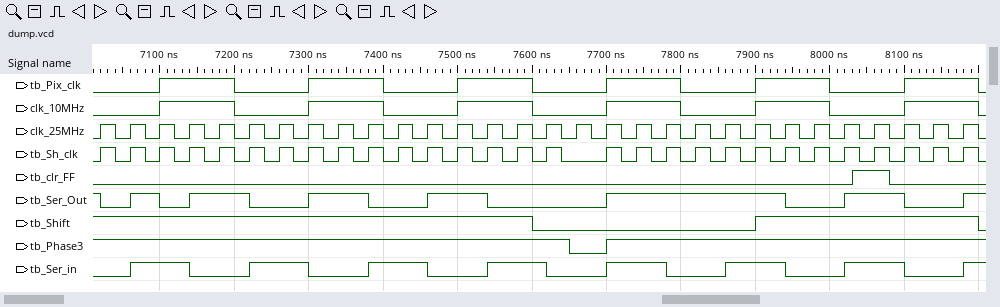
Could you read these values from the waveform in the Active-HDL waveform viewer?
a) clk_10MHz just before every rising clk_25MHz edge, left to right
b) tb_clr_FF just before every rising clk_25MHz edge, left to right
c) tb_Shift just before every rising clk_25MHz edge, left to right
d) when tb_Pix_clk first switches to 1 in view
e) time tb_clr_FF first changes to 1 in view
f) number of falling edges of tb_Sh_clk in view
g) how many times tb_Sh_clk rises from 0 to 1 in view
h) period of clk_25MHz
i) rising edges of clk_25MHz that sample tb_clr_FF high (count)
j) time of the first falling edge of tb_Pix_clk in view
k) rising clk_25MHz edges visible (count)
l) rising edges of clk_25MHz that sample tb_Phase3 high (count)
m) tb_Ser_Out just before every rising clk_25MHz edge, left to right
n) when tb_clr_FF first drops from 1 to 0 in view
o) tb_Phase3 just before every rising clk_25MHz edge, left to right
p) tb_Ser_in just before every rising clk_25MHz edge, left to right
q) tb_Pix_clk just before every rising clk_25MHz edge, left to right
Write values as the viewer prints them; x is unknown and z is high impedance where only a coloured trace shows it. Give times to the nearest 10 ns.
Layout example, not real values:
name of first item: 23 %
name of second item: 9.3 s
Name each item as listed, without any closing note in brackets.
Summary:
clk_10MHz just before every rising clk_25MHz edge, left to right: 0 0 0 1 1 0 0 0 1 1 0 0 0 1 1 0 0 0 1 1 0 0 0 1 1 0 0 0 1 1
tb_clr_FF just before every rising clk_25MHz edge, left to right: 0 0 0 0 0 0 0 0 0 0 0 0 0 0 0 0 0 0 0 0 0 0 0 0 0 0 1 0 0 0
tb_Shift just before every rising clk_25MHz edge, left to right: 1 1 1 1 1 1 1 1 1 1 1 1 1 1 1 0 0 0 0 0 0 0 0 1 1 1 1 1 1 1
when tb_Pix_clk first switches to 1 in view: 7100 ns
time tb_clr_FF first changes to 1 in view: 8030 ns
number of falling edges of tb_Sh_clk in view: 29
how many times tb_Sh_clk rises from 0 to 1 in view: 29
period of clk_25MHz: 40 ns
rising edges of clk_25MHz that sample tb_clr_FF high: 1
time of the first falling edge of tb_Pix_clk in view: 7200 ns
rising clk_25MHz edges visible: 30
rising edges of clk_25MHz that sample tb_Phase3 high: 28
tb_Ser_Out just before every rising clk_25MHz edge, left to right: 1 0 1 0 1 1 0 0 1 1 0 0 1 1 0 0 0 0 1 1 1 1 1 1 0 0 1 1 0 0
when tb_clr_FF first drops from 1 to 0 in view: 8080 ns
tb_Phase3 just before every rising clk_25MHz edge, left to right: 1 1 1 1 1 1 1 1 1 1 1 1 1 1 1 1 0 0 1 1 1 1 1 1 1 1 1 1 1 1
tb_Ser_in just before every rising clk_25MHz edge, left to right: 0 0 1 1 0 0 1 1 0 0 1 1 0 0 1 1 0 0 1 1 0 0 1 1 0 0 1 1 0 0
tb_Pix_clk just before every rising clk_25MHz edge, left to right: 0 0 0 1 1 0 0 0 1 1 0 0 0 1 1 0 0 0 1 1 0 0 0 1 1 0 0 0 1 1
